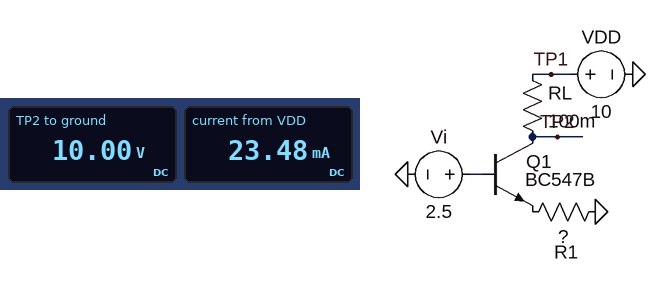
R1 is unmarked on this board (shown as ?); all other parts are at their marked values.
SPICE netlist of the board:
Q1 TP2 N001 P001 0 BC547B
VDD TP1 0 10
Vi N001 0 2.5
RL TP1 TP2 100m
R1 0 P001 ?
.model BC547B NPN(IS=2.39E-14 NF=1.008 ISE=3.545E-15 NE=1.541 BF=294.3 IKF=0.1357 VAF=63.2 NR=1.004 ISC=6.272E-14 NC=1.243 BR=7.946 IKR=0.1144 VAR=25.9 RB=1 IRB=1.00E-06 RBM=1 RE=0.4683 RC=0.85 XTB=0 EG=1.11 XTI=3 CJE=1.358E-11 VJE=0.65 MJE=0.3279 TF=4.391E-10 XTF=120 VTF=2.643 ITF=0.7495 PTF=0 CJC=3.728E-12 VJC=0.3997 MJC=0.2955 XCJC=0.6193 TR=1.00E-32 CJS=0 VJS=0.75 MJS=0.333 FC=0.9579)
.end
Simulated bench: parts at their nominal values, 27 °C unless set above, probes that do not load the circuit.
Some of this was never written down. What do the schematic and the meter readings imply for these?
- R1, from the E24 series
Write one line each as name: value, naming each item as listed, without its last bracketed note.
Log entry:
R1, from the E24 series: 75 Ω
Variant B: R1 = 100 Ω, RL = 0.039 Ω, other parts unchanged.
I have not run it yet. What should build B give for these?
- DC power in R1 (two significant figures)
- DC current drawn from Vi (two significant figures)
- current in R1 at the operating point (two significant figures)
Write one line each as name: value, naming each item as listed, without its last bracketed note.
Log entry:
DC power in R1: 32 mW
DC current drawn from Vi: 62 µA
current in R1 at the operating point: 18 mA
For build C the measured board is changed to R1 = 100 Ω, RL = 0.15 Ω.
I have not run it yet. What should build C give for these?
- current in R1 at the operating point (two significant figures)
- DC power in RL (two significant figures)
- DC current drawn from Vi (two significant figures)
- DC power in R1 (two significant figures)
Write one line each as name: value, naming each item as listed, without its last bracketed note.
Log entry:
current in R1 at the operating point: 18 mA
DC power in RL: 47 µW
DC current drawn from Vi: 62 µA
DC power in R1: 32 mW
